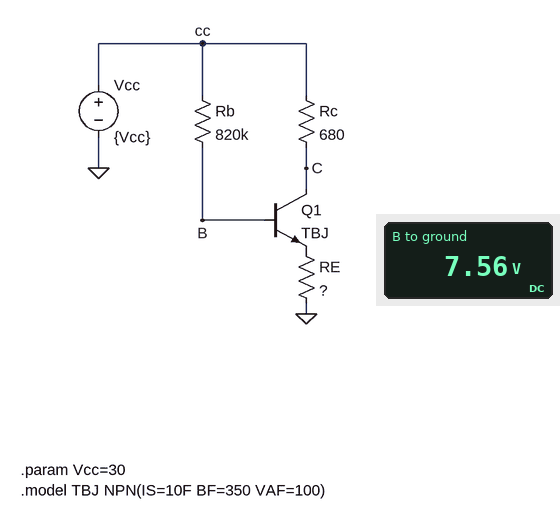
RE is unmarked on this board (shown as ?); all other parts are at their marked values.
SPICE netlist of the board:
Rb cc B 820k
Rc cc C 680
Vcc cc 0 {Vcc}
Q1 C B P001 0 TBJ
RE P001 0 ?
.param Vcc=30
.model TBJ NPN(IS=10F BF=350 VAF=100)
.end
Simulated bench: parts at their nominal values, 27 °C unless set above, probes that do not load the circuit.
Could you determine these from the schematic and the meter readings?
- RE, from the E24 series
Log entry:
620 Ω
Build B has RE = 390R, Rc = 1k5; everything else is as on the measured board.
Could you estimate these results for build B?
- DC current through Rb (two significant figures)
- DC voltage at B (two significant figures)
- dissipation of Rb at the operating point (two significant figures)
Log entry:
30 µA
5.2 V
750 µW
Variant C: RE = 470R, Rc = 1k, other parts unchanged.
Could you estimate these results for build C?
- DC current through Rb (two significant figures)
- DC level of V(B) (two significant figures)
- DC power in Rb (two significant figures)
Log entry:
29 µA
6.1 V
700 µW
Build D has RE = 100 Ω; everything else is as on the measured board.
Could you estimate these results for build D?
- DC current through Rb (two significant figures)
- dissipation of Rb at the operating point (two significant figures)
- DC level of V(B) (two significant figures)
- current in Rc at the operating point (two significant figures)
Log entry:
34 µA
950 µW
2.1 V
14 mA
